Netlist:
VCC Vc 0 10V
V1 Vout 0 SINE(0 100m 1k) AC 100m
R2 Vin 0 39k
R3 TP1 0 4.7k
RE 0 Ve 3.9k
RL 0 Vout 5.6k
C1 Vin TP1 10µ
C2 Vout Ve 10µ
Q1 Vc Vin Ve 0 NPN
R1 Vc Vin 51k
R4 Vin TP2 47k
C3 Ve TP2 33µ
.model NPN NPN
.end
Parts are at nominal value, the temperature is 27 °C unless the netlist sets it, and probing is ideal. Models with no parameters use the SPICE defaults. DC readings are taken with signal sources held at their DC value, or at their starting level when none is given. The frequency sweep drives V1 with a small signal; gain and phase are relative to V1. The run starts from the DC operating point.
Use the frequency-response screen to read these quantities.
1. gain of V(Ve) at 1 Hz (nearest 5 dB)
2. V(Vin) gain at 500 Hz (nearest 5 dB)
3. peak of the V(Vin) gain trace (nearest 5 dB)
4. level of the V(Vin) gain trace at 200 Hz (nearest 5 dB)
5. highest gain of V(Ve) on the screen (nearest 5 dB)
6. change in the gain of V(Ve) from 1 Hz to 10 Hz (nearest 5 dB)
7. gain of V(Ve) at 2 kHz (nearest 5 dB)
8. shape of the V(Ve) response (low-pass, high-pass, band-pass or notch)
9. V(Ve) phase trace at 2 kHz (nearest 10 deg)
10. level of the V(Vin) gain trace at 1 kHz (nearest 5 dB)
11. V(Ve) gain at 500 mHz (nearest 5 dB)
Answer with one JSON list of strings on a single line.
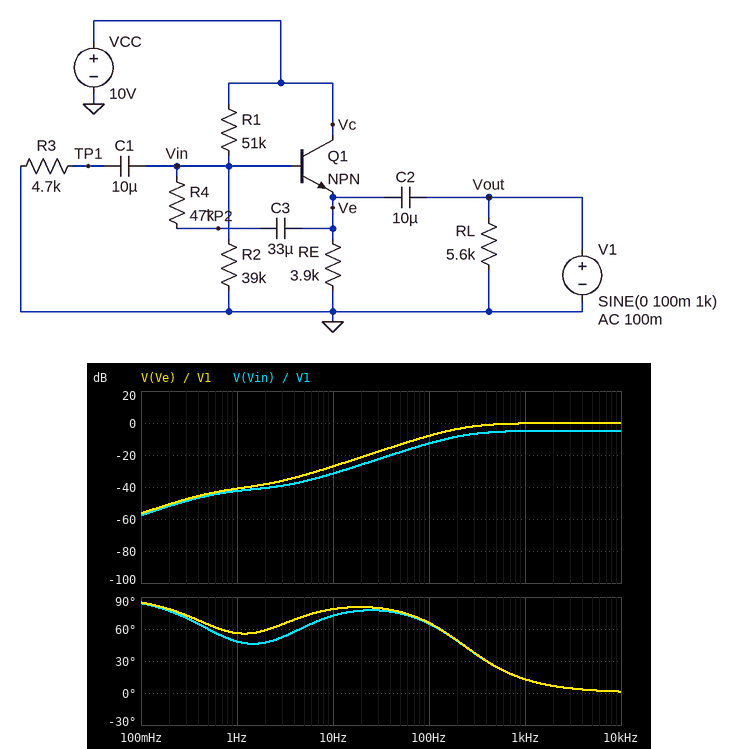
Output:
["-40 dB", "-5 dB", "-5 dB", "-10 dB", "0 dB", "15 dB", "0 dB", "high-pass", "10 deg", "-5 dB", "-45 dB"]
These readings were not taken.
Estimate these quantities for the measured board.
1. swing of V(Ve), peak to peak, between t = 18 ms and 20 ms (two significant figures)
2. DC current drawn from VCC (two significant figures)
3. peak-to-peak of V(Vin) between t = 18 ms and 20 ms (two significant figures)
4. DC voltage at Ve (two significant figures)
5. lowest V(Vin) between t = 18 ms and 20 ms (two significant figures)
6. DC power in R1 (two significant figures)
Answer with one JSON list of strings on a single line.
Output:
["200 mV", "970 µA", "92 mV", "3.4 V", "4.1 V", "670 µW"]
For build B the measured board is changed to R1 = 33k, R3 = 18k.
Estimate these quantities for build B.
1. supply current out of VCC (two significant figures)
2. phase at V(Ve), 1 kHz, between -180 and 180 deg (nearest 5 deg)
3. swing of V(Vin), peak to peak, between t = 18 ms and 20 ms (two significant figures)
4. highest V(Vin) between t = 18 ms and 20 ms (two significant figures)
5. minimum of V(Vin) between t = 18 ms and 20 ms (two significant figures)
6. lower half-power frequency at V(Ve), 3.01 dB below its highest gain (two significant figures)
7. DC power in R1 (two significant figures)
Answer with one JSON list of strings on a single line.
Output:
["1.3 mA", "10 deg", "150 mV", "5.3 V", "5.1 V", "140 Hz", "690 µW"]
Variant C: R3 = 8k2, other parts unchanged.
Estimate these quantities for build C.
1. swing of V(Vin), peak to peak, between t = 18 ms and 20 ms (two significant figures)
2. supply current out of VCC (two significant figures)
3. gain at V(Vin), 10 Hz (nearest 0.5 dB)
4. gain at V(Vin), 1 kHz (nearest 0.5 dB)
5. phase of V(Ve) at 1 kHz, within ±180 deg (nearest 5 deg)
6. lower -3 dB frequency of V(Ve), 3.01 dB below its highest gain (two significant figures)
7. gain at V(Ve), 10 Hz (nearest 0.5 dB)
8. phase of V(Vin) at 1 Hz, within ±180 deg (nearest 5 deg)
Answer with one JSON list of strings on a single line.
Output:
["120 mV", "970 µA", "-28.0 dB", "-3.5 dB", "10 deg", "180 Hz", "-25.0 dB", "55 deg"]
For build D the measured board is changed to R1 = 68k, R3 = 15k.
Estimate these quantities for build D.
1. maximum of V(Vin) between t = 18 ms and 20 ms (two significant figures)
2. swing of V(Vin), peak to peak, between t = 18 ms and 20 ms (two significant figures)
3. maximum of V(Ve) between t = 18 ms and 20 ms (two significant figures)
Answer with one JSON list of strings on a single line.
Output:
["3.5 V", "130 mV", "2.8 V"]
